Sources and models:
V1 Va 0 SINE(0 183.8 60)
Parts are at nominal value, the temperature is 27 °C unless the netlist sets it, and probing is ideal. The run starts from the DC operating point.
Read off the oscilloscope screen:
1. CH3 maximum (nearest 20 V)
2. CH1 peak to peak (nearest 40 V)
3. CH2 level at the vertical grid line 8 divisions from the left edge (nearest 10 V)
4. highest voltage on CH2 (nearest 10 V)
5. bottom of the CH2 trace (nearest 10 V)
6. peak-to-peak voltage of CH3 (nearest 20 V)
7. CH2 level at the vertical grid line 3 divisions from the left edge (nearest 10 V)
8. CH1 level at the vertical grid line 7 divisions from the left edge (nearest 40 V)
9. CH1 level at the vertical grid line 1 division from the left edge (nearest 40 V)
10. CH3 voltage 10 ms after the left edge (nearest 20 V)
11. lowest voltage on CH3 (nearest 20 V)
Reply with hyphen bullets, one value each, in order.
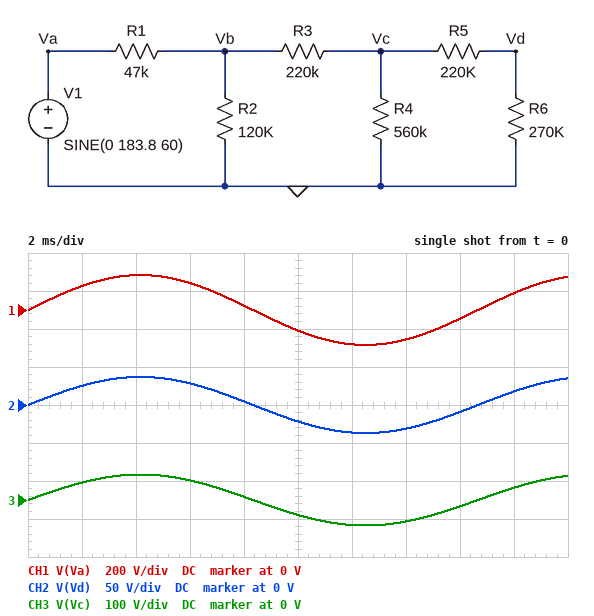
- 60 V
- 360 V
- -10 V
- 40 V
- -40 V
- 140 V
- 30 V
- -160 V
- 120 V
- -40 V
- -60 V
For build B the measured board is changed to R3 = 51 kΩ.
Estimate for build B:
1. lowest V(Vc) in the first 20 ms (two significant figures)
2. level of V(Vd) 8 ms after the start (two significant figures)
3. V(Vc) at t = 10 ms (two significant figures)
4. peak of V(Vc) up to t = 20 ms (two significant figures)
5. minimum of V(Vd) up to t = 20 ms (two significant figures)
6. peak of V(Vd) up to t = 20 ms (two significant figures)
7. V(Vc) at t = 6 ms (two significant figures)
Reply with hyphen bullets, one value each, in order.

- -100 V
- 6.9 V
- -59 V
- 100 V
- -55 V
- 55 V
- 77 V
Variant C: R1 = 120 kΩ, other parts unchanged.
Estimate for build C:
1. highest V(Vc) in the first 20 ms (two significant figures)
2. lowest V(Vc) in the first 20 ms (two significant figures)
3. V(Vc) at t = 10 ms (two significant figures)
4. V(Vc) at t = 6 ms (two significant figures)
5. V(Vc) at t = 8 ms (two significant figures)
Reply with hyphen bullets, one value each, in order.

- 44 V
- -44 V
- -26 V
- 34 V
- 5.6 V
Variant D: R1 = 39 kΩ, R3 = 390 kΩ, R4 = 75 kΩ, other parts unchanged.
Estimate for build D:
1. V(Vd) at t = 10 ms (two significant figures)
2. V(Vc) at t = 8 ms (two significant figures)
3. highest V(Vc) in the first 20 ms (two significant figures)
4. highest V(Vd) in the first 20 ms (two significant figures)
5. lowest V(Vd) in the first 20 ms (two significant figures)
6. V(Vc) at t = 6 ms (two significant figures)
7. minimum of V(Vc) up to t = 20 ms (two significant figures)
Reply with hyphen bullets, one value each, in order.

- -6.0 V
- 2.3 V
- 19 V
- 10 V
- -10 V
- 14 V
- -19 V
